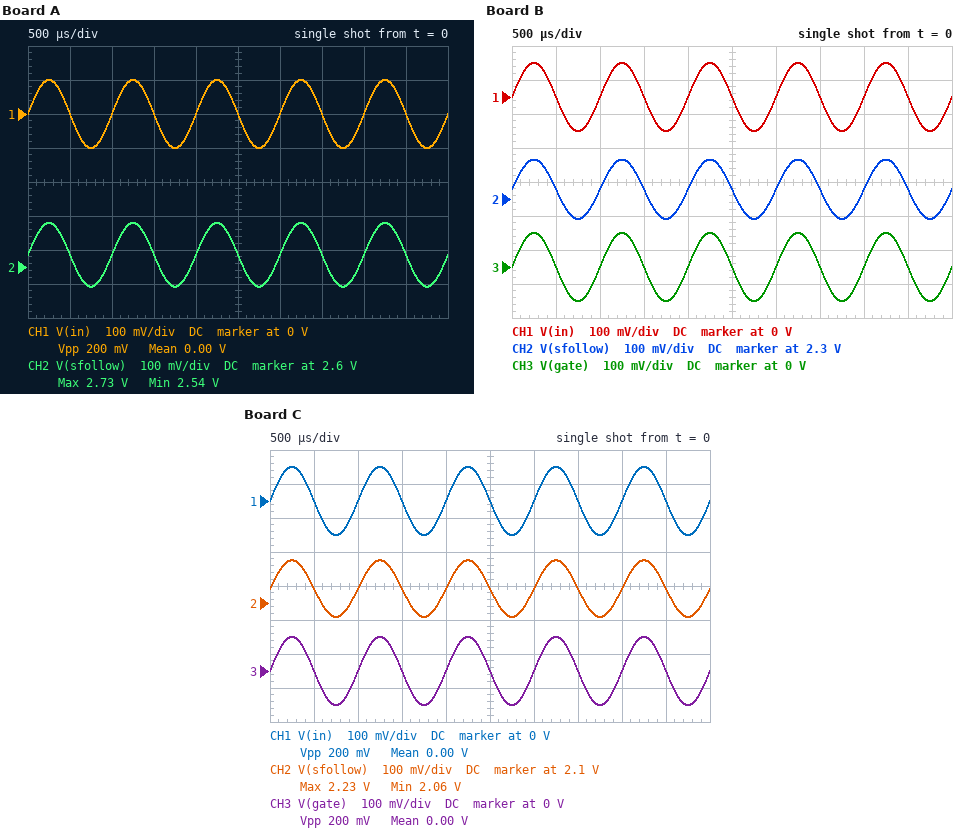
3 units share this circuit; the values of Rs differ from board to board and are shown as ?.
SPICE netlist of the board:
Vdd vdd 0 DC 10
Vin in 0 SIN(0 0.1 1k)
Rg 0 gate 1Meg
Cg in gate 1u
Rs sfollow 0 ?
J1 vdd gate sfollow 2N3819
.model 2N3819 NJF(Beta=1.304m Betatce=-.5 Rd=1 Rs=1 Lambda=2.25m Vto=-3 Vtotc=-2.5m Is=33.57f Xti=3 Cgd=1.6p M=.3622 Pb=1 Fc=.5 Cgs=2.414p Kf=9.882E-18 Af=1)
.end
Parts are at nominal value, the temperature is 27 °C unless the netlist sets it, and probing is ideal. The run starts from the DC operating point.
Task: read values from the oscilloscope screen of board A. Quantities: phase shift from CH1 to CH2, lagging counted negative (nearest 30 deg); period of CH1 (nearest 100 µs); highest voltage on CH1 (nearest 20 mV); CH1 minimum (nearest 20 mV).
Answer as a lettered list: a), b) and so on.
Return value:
a) 0 deg
b) 1.0 ms
c) 100 mV
d) -100 mV
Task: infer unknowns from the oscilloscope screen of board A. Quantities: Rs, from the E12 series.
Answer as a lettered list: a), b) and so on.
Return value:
a) 15 kΩ
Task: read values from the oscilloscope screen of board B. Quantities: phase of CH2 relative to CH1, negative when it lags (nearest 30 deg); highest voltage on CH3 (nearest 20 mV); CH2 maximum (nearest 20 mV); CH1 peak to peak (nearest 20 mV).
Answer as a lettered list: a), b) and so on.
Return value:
a) 0 deg
b) 100 mV
c) 2.42 V
d) 200 mV
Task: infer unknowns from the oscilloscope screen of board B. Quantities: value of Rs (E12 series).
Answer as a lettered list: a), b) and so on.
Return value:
a) 3.9 kΩ
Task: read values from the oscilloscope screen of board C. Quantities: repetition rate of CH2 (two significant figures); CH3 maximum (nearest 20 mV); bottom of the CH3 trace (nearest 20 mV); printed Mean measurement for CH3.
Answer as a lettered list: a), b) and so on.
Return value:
a) 1.0 kHz
b) 100 mV
c) -100 mV
d) 0.00 V
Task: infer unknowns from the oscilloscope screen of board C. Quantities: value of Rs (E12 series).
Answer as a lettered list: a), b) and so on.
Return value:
a) 2.2 kΩ
